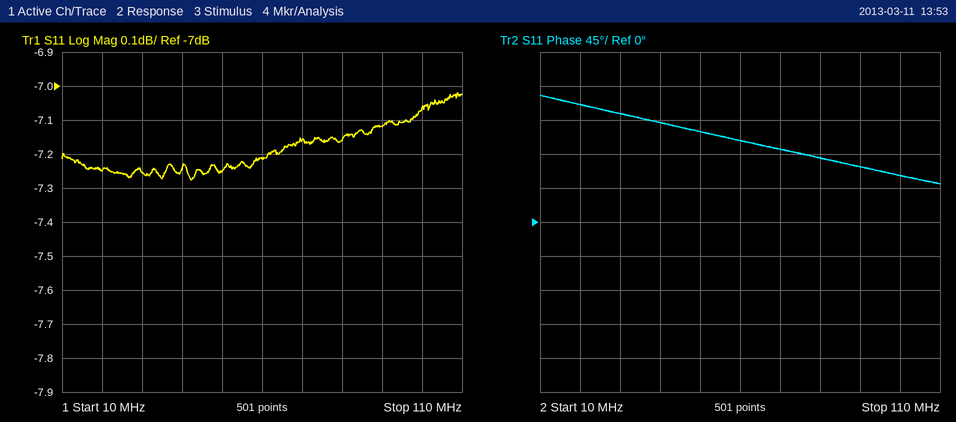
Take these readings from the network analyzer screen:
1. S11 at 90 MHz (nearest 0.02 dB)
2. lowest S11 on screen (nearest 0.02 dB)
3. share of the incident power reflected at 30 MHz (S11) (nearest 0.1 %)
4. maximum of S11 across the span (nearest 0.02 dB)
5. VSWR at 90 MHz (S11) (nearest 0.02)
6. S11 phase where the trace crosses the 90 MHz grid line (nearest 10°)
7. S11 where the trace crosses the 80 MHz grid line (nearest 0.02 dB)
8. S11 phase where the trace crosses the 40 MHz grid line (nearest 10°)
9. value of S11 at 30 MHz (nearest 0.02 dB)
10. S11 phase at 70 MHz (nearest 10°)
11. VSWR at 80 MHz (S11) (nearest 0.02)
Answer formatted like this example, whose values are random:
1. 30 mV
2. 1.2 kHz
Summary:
1. -7.12 dB
2. -7.28 dB
3. 18.8 %
4. -7.02 dB
5. 2.58
6. 70°
7. -7.16 dB
8. 130°
9. -7.26 dB
10. 100°
11. 2.56
